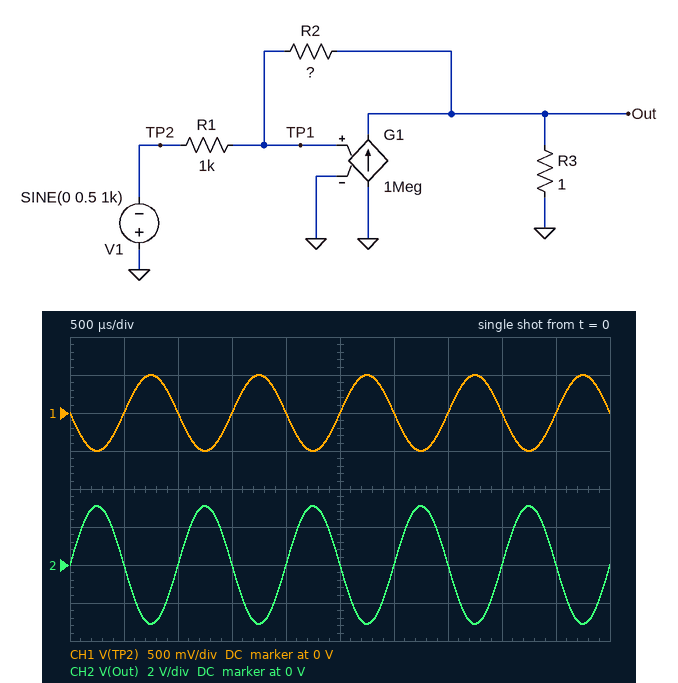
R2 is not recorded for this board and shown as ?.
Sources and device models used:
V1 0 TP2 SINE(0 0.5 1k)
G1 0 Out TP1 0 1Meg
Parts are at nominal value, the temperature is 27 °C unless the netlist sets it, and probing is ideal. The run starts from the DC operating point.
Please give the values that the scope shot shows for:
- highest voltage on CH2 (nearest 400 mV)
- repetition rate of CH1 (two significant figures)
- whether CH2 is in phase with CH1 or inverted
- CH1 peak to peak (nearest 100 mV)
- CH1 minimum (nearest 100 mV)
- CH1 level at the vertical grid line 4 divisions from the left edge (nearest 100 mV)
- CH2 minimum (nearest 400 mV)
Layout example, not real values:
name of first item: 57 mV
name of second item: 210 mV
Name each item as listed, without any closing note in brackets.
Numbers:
highest voltage on CH2: 3.2 V
repetition rate of CH1: 1.0 kHz
whether CH2 is in phase with CH1 or inverted: inverted
CH1 peak to peak: 1.0 V
CH1 minimum: -500 mV
CH1 level at the vertical grid line 4 divisions from the left edge: 0 V
CH2 minimum: -3.2 V
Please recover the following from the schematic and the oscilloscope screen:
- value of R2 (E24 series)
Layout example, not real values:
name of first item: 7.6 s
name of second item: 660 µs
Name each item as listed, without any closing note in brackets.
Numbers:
value of R2: 6.2 kΩ
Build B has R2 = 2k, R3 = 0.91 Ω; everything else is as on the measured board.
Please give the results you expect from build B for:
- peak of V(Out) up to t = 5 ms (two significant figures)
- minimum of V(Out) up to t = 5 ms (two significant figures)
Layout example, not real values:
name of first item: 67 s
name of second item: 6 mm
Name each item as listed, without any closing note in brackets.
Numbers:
peak of V(Out) up to t = 5 ms: 1.0 V
minimum of V(Out) up to t = 5 ms: -1.0 V
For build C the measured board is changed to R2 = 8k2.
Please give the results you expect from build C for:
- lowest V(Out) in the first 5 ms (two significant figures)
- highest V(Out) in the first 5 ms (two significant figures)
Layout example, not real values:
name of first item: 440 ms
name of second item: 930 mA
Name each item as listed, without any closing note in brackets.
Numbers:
lowest V(Out) in the first 5 ms: -4.1 V
highest V(Out) in the first 5 ms: 4.1 V
